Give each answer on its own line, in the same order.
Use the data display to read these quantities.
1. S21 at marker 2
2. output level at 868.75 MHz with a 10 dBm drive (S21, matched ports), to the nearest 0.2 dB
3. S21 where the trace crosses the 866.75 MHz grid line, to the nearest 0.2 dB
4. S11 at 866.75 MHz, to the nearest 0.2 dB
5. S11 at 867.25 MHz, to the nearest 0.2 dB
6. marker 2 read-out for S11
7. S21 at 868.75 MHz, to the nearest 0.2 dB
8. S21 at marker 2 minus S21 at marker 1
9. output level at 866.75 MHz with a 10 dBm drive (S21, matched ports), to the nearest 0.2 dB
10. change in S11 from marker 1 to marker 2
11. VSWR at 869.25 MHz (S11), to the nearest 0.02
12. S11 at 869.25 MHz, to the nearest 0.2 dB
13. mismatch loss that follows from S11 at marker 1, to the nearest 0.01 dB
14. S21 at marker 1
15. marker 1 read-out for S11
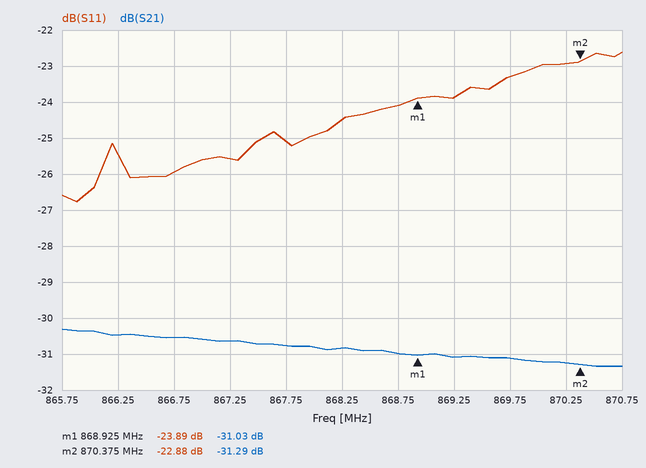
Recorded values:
-31.29 dB
-21.0 dBm
-30.6 dB
-26.0 dB
-25.6 dB
-22.88 dB
-31.0 dB
-0.26 dB
-20.6 dBm
1.01 dB
1.14
-23.8 dB
0.02 dB
-31.03 dB
-23.89 dB
